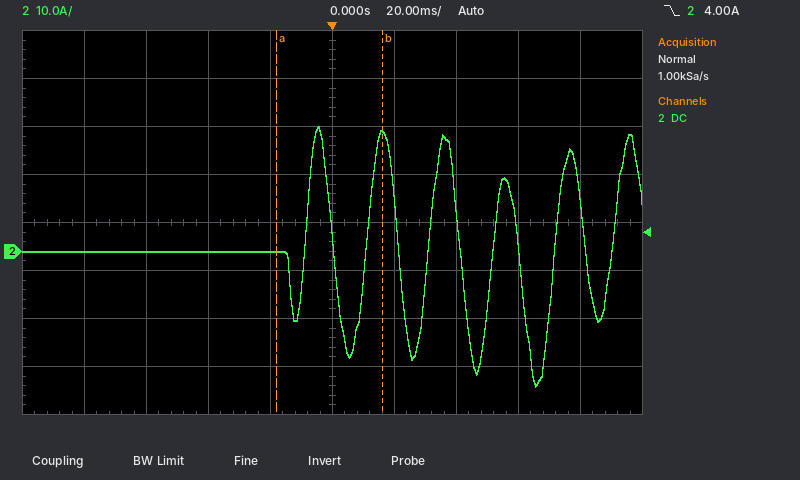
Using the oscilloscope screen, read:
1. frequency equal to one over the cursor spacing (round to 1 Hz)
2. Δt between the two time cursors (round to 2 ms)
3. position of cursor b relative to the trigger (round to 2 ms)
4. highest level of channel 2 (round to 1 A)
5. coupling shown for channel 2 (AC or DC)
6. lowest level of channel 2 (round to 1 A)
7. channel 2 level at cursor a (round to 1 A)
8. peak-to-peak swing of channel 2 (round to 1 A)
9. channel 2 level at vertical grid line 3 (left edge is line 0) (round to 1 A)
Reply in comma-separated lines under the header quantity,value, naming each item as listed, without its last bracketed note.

quantity,value
frequency equal to one over the cursor spacing,29 Hz
Δt between the two time cursors,34 ms
position of cursor b relative to the trigger,+16 ms
highest level of channel 2,26 A
coupling shown for channel 2,DC
lowest level of channel 2,-28 A
channel 2 level at cursor a,0 A
peak-to-peak swing of channel 2,54 A
channel 2 level at vertical grid line 3 (left edge is line 0),0 A
